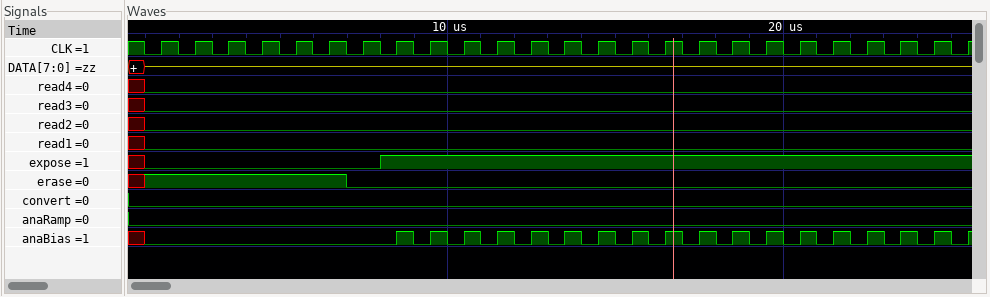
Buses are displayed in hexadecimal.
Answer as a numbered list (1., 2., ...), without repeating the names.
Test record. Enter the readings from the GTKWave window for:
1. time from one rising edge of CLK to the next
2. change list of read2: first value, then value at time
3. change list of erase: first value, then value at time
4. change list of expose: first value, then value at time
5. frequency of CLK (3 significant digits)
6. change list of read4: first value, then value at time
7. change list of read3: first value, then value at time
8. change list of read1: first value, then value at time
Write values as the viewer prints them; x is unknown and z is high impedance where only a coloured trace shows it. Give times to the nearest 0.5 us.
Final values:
1. 1 us
2. x, 0 at 1 us
3. x, 1 at 1 us, 0 at 7 us
4. x, 0 at 1 us, 1 at 8 us
5. 1.00 MHz
6. x, 0 at 1 us
7. x, 0 at 1 us
8. x, 0 at 1 us
